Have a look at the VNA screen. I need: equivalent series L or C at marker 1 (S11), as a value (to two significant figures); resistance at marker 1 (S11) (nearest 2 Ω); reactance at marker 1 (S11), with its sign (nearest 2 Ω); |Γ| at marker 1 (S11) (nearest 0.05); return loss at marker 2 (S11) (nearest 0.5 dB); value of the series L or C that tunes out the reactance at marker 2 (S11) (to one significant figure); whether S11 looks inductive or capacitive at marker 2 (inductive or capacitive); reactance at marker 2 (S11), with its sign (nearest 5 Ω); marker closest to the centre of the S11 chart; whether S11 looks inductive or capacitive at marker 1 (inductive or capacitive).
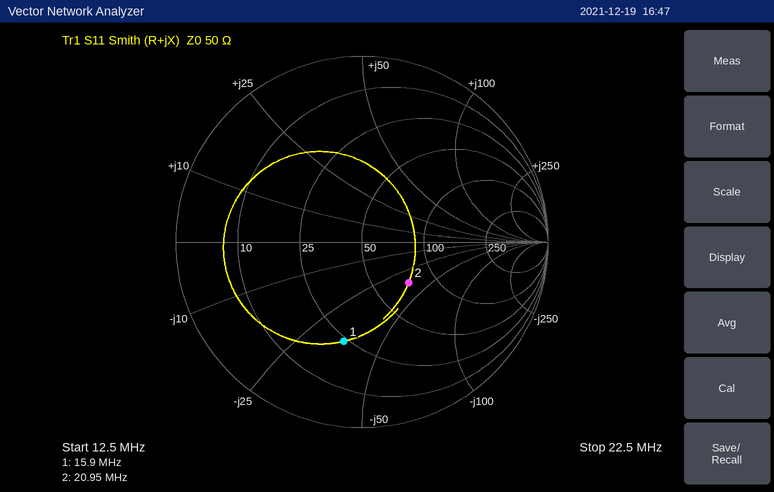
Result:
280 pF
24 Ω
-36 Ω
0.55
9.5 dB
300 nH
capacitive
-35 Ω
marker 2
capacitive
